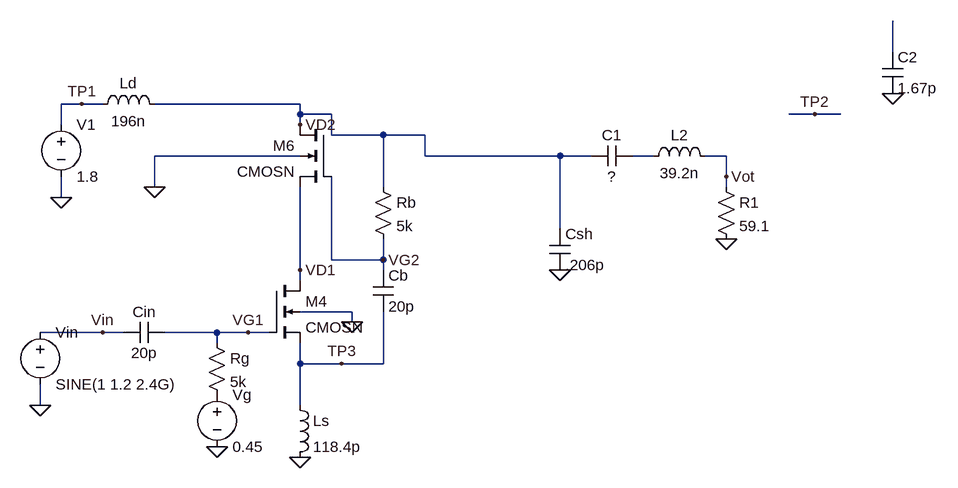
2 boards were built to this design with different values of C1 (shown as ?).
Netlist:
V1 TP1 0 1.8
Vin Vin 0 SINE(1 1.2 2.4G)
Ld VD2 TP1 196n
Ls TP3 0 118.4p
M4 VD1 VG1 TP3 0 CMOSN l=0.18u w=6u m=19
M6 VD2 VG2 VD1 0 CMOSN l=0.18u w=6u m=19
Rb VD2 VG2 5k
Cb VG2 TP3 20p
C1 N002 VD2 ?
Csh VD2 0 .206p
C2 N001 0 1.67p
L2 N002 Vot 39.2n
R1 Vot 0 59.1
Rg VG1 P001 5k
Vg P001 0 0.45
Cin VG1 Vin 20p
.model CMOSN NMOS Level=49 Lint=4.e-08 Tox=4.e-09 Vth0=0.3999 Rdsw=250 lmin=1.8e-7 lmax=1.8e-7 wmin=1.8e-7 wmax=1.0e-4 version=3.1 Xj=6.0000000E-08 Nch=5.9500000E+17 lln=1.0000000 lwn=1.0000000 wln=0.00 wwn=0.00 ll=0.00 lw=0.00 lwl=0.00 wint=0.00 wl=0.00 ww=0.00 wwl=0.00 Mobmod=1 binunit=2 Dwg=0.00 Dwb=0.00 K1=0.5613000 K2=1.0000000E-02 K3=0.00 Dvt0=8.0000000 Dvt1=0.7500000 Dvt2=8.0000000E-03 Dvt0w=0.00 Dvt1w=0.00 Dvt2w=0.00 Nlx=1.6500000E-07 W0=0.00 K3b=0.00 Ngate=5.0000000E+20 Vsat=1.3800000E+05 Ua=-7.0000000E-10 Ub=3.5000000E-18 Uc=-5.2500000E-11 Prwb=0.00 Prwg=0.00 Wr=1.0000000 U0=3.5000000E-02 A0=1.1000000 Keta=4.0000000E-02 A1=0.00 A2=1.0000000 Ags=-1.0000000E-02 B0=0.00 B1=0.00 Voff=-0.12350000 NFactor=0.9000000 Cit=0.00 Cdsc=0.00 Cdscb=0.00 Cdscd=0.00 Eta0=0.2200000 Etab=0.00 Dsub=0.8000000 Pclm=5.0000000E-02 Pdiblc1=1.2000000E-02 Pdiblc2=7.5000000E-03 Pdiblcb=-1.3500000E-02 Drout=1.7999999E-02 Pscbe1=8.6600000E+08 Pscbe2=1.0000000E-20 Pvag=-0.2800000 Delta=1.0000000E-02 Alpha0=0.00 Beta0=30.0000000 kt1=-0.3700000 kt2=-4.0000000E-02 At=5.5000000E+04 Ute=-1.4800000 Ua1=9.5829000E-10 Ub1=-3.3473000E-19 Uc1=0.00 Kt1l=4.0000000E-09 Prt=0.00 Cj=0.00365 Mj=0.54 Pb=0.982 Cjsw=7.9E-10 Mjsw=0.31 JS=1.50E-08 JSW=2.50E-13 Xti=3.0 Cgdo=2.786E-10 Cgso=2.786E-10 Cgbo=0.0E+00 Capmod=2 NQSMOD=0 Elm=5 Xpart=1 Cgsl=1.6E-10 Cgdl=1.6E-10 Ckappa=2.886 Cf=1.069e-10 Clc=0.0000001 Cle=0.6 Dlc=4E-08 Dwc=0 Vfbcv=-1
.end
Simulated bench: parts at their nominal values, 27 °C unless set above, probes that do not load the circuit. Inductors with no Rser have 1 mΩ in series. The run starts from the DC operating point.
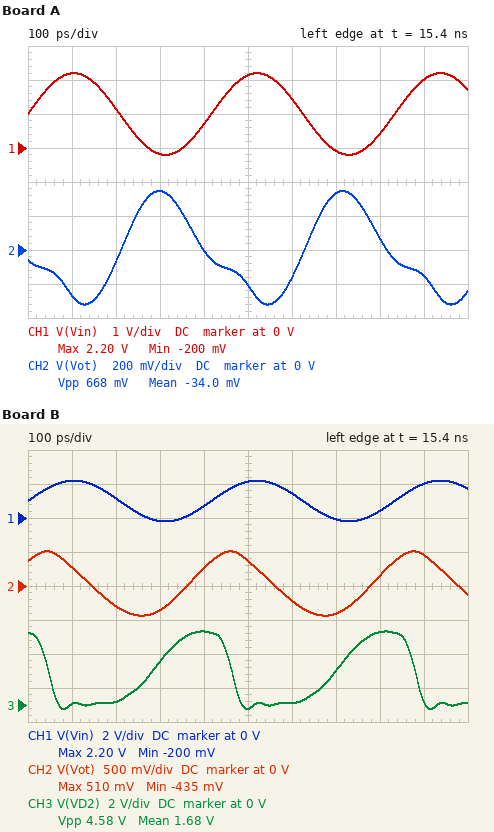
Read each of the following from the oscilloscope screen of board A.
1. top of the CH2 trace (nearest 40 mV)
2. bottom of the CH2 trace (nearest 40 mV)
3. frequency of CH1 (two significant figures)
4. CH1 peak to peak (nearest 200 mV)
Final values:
360 mV
-320 mV
2.4 GHz
2.4 V
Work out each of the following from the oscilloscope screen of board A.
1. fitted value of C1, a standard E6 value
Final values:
68 fF
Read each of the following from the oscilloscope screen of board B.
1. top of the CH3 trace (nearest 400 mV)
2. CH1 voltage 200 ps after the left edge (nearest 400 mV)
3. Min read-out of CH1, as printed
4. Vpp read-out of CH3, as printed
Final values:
4.4 V
1.2 V
-200 mV
4.58 V
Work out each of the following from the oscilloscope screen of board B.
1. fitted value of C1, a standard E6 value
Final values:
220 fF
